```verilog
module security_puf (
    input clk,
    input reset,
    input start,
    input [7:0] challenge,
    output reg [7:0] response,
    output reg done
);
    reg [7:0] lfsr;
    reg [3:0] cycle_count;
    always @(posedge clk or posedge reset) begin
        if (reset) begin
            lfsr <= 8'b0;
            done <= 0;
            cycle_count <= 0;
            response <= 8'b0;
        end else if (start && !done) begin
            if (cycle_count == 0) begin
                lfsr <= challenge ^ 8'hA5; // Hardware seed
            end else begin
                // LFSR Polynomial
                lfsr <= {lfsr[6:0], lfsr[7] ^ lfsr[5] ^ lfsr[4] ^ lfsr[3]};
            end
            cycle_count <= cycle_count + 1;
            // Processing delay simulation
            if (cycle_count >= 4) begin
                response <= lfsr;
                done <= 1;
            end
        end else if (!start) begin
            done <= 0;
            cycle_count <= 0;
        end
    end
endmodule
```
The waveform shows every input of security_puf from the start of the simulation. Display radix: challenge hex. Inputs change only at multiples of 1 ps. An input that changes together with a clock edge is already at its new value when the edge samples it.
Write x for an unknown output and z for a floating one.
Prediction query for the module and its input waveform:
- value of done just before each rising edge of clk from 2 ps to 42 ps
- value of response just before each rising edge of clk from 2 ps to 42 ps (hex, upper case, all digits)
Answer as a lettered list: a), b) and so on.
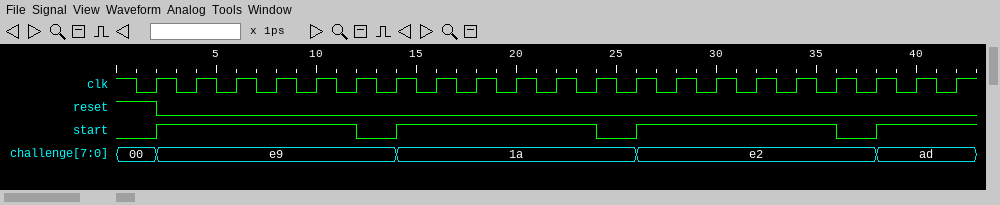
a) 0 0 0 0 0 1 0 0 0 0 0 1 0 0 0 0 0 1 0 0 0
b) 00, 00, 00, 00, 00, 66, 66, 66, 66, 66, 66, FA, FA, FA, FA, FA, FA, 38, 38, 38, 38
